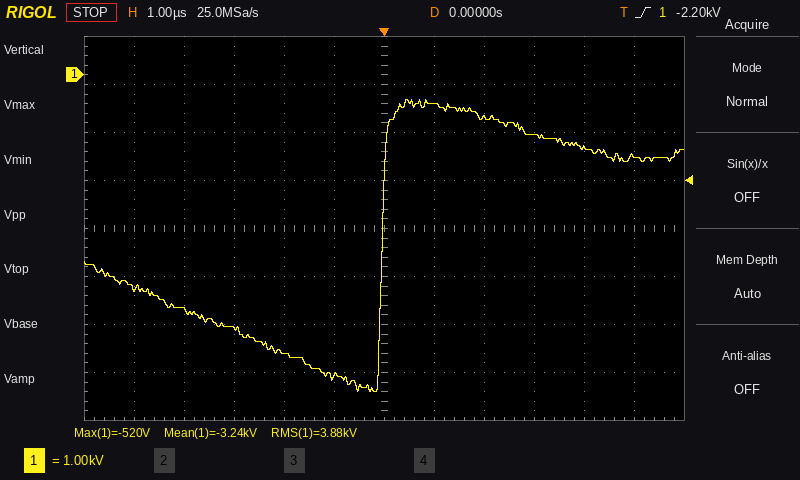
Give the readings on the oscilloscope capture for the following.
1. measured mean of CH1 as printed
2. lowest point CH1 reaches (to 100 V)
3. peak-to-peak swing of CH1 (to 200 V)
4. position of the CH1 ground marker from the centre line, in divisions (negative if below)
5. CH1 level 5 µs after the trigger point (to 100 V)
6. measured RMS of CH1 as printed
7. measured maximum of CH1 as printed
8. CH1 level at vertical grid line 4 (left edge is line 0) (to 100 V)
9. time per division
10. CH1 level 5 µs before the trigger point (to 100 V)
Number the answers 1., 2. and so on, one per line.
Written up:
1. -3.24 kV
2. -6.6 kV
3. 6.0 kV
4. +3.2 div
5. -1.7 kV
6. 3.88 kV
7. -520 V
8. -5.8 kV
9. 1 µs
10. -4.4 kV
